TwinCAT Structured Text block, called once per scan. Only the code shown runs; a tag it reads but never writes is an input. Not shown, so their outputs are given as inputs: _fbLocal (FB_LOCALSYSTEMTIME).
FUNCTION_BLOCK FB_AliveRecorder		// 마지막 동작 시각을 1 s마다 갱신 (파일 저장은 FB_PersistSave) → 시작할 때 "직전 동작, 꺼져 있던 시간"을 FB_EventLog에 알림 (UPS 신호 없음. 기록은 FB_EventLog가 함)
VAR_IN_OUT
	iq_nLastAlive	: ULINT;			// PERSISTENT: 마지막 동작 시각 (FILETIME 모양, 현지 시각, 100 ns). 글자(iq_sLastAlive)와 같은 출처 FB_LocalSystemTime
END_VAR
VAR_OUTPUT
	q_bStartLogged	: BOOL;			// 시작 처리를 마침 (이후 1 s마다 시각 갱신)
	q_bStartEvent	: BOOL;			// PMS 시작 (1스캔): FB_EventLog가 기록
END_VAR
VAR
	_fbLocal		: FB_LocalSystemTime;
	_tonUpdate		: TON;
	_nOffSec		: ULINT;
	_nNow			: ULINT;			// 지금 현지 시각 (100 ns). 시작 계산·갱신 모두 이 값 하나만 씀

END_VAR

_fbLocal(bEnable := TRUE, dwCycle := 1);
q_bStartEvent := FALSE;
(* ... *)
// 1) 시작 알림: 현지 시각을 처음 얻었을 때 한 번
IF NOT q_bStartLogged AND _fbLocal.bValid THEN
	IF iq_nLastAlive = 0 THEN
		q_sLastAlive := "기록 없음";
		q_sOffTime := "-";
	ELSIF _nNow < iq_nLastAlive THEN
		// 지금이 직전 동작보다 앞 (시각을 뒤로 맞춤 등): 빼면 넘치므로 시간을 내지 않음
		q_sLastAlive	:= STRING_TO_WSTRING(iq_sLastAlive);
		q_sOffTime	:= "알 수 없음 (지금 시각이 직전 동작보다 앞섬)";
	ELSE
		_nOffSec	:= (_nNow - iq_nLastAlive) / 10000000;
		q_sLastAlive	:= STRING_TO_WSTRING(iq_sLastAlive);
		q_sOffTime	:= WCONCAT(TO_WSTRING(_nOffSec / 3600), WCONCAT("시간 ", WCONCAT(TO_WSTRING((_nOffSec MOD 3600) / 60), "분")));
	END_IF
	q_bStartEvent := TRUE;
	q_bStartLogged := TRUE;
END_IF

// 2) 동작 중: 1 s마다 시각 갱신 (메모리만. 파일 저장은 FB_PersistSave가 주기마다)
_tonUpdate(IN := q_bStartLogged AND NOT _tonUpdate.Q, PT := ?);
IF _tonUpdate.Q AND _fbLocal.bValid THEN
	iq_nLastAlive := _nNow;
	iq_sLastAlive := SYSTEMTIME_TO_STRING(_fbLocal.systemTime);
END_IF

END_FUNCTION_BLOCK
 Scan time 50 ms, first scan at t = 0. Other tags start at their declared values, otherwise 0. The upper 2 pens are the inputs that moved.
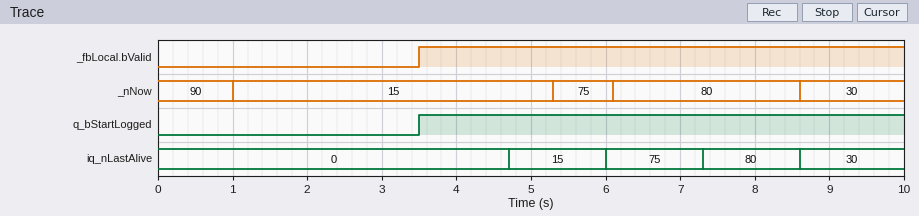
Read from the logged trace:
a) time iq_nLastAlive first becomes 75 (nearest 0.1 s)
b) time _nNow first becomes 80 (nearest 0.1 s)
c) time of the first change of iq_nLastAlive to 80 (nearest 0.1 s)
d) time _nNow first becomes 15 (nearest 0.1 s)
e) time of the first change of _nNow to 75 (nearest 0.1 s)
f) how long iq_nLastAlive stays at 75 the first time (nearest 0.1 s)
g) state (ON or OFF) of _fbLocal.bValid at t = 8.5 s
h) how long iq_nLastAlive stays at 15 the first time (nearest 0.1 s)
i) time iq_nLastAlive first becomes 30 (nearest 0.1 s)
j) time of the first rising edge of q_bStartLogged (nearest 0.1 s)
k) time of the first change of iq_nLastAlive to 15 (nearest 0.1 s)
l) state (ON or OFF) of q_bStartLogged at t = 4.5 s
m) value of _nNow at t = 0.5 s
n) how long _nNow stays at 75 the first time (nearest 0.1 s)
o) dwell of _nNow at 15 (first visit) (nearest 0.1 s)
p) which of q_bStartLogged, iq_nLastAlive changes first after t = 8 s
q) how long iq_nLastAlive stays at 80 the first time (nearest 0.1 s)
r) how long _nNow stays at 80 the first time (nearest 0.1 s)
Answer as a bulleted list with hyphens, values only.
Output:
- 6.0 s
- 6.1 s
- 7.3 s
- 1.0 s
- 5.3 s
- 1.3 s
- ON
- 1.3 s
- 8.6 s
- 3.5 s
- 4.7 s
- ON
- 90
- 0.8 s
- 4.3 s
- iq_nLastAlive
- 1.3 s
- 2.5 s
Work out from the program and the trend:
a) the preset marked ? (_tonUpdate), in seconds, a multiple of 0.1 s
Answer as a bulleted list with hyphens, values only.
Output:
- 1.2 s
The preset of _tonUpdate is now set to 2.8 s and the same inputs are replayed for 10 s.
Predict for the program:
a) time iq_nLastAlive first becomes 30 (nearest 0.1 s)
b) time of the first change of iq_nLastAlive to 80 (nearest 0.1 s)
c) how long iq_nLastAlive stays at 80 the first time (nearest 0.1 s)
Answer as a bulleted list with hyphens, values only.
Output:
- 9.2 s
- 6.3 s
- 2.9 s
